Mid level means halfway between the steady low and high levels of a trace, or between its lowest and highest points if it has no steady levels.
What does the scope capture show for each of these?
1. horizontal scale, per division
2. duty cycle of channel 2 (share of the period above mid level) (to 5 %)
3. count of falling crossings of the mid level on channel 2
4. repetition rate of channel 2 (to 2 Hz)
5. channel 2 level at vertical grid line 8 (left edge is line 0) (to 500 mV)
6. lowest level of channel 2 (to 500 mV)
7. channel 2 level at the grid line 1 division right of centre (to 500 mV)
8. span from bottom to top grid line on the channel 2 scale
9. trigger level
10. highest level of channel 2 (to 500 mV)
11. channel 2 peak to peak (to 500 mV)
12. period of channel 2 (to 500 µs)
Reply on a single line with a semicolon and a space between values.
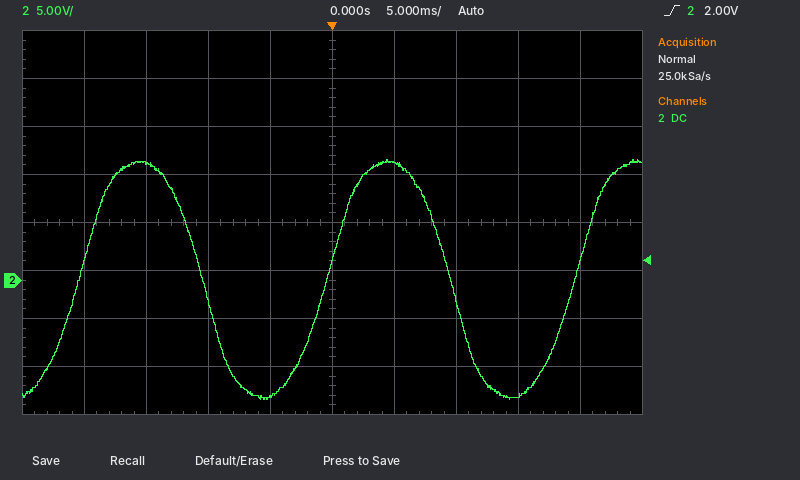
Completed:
5 ms; 50 %; 2; 50 Hz; -12.0 V; -12.5 V; 12.0 V; 40 V; 2.00 V; 12.5 V; 25.0 V; 20.0 ms
